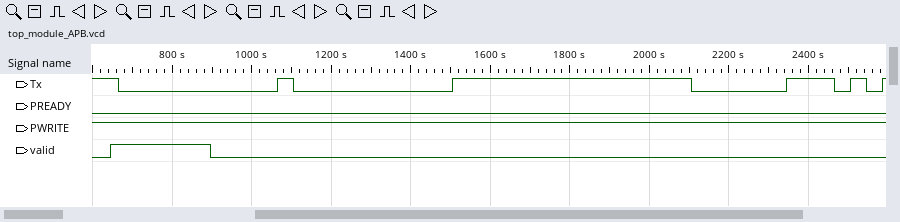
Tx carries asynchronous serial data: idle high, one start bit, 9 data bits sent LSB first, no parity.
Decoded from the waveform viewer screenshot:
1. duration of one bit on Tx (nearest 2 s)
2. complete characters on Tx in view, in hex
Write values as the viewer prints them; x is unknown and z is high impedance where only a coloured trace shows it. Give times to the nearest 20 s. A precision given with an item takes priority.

40 s
00, 00, E0
